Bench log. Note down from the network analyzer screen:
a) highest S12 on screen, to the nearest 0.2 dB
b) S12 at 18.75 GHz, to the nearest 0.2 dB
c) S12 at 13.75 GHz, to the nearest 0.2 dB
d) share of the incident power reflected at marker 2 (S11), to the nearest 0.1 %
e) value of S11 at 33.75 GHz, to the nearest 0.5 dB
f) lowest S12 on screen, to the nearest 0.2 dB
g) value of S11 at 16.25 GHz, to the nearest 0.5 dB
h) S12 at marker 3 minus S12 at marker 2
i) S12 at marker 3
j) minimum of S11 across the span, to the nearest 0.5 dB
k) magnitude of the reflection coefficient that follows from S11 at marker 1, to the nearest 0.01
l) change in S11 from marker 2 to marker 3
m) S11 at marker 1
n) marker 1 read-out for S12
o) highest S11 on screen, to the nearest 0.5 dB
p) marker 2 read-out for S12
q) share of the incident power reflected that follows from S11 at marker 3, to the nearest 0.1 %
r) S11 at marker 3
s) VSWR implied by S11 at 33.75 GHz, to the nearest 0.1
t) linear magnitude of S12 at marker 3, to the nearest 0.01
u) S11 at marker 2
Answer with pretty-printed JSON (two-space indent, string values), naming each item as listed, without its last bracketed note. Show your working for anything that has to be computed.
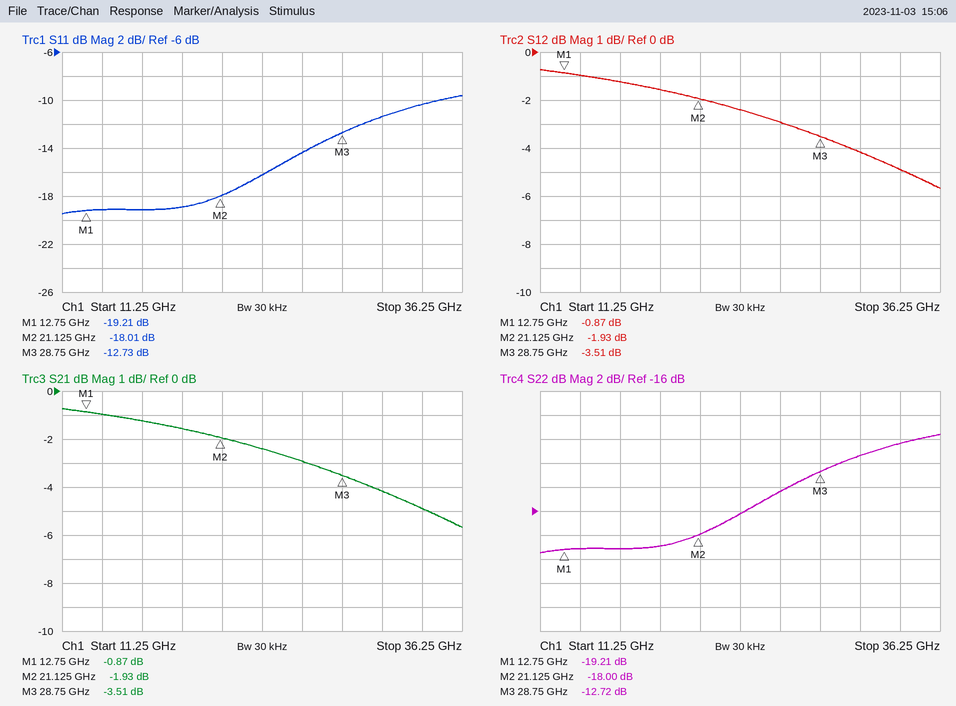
{
  "highest S12 on screen, to the nearest 0.2 dB": "-0.8 dB",
  "S12 at 18.75 GHz, to the nearest 0.2 dB": "-1.6 dB",
  "S12 at 13.75 GHz, to the nearest 0.2 dB": "-1.0 dB",
  "share of the incident power reflected at marker 2 (S11), to the nearest 0.1 %": "10^(-18.01/10) ≈ 1.6 %",
  "value of S11 at 33.75 GHz, to the nearest 0.5 dB": "-10.5 dB",
  "lowest S12 on screen, to the nearest 0.2 dB": "-5.6 dB",
  "value of S11 at 16.25 GHz, to the nearest 0.5 dB": "-19.0 dB",
  "S12 at marker 3 minus S12 at marker 2": "-3.51 − (-1.93) = -1.58 dB",
  "S12 at marker 3": "-3.51 dB",
  "minimum of S11 across the span, to the nearest 0.5 dB": "-19.5 dB",
  "magnitude of the reflection coefficient that follows from S11 at marker 1, to the nearest 0.01": "10^(-19.21/20) ≈ 0.11",
  "change in S11 from marker 2 to marker 3": "-12.73 − (-18.01) = 5.28 dB",
  "S11 at marker 1": "-19.21 dB",
  "marker 1 read-out for S12": "-0.87 dB",
  "highest S11 on screen, to the nearest 0.5 dB": "-9.5 dB",
  "marker 2 read-out for S12": "-1.93 dB",
  "share of the incident power reflected that follows from S11 at marker 3, to the nearest 0.1 %": "10^(-12.73/10) ≈ 5.3 %",
  "S11 at marker 3": "-12.73 dB",
  "VSWR implied by S11 at 33.75 GHz, to the nearest 0.1": "|Γ| = 10^(-10.5/20) = 0.2985; VSWR = (1 + 0.2985)/(1 − 0.2985) ≈ 1.9",
  "linear magnitude of S12 at marker 3, to the nearest 0.01": "10^(-3.51/20) ≈ 0.67",
  "S11 at marker 2": "-18.01 dB"
}
